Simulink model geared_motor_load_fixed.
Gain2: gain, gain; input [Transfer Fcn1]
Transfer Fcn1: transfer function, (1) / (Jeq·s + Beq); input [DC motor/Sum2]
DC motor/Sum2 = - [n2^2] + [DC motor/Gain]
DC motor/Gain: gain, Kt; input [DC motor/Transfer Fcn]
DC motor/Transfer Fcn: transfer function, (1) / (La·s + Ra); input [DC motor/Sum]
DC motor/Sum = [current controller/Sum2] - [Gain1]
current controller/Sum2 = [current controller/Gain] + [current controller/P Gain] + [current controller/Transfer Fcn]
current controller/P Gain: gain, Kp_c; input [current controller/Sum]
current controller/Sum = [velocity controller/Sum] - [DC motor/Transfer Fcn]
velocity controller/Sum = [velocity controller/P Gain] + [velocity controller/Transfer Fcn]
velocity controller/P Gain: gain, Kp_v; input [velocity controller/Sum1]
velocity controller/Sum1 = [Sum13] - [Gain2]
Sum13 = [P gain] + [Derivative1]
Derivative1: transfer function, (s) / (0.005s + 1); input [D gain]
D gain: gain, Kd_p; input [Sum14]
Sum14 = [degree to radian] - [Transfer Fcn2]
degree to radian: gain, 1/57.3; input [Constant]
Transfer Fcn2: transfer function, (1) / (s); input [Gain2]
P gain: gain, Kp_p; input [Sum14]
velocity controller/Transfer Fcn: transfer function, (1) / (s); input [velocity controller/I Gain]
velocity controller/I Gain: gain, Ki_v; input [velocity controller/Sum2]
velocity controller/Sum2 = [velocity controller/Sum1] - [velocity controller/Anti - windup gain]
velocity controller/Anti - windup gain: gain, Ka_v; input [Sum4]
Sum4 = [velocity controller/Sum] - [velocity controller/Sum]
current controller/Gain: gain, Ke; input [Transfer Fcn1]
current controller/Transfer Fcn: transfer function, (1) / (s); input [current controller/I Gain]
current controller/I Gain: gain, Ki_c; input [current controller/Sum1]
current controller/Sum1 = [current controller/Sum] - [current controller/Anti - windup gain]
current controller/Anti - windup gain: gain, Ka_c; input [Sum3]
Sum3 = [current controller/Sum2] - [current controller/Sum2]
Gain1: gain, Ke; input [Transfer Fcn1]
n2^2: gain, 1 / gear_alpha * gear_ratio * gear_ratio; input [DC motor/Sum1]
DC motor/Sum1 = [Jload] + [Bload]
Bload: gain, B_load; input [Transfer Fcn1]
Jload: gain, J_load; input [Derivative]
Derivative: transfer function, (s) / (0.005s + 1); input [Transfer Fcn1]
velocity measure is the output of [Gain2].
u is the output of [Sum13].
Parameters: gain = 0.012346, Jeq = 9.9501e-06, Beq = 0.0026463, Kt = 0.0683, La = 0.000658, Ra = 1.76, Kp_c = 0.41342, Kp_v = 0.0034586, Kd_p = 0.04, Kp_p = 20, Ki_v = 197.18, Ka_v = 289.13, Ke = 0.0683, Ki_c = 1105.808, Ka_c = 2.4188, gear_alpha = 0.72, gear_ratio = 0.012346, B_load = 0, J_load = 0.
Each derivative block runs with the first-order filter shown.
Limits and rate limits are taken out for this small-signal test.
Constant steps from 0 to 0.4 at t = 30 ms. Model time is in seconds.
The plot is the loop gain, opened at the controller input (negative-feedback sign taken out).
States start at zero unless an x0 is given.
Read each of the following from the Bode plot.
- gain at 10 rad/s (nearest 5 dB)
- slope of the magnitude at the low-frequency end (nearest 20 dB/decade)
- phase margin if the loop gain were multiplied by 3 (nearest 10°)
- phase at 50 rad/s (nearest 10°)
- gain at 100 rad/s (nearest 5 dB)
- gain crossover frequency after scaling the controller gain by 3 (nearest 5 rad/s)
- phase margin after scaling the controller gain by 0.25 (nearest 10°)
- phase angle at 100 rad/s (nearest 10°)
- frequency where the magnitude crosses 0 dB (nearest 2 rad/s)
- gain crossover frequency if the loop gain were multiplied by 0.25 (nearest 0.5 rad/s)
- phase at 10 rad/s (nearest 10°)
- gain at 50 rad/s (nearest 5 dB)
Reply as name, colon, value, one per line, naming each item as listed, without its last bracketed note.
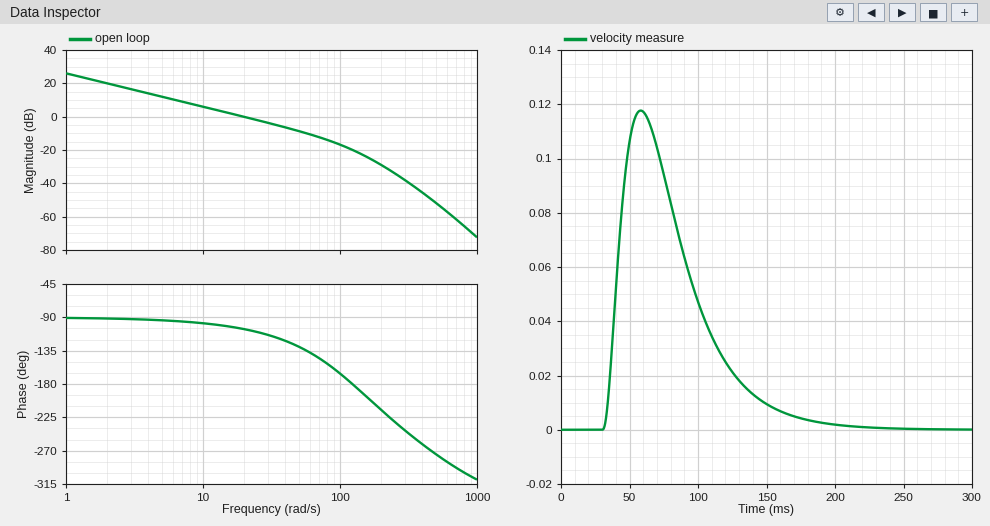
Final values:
gain at 10 rad/s: 5 dB
slope of the magnitude at the low-frequency end: -20 dB/decade
phase margin if the loop gain were multiplied by 3: 50°
phase at 50 rad/s: -130°
gain at 100 rad/s: -15 dB
gain crossover frequency after scaling the controller gain by 3: 55 rad/s
phase margin after scaling the controller gain by 0.25: 90°
phase angle at 100 rad/s: -170°
frequency where the magnitude crosses 0 dB: 20 rad/s
gain crossover frequency if the loop gain were multiplied by 0.25: 5.0 rad/s
phase at 10 rad/s: -100°
gain at 50 rad/s: -10 dB
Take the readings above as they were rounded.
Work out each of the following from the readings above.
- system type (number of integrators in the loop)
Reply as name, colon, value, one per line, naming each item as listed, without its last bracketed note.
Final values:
system type: 1
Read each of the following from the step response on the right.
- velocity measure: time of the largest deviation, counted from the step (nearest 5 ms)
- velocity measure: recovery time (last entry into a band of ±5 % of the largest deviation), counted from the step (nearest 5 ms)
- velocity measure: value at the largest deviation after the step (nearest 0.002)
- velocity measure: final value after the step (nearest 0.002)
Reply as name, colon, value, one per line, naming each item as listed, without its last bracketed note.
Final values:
velocity measure: time of the largest deviation, counted from the step: 30 ms
velocity measure: recovery time (last entry into a band of ±5 % of the largest deviation), counted from the step: 135 ms
velocity measure: value at the largest deviation after the step: 0.118
velocity measure: final value after the step: 0.000
